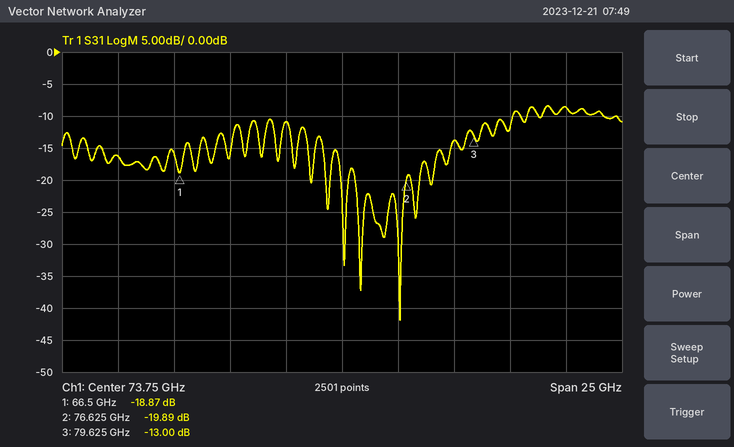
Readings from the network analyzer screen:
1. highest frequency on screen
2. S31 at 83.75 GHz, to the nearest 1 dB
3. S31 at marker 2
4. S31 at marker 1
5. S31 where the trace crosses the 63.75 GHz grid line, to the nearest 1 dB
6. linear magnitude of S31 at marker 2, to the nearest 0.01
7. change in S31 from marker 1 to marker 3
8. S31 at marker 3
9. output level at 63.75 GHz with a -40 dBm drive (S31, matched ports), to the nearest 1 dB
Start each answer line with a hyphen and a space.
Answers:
- 86.25 GHz
- -9 dB
- -19.89 dB
- -18.87 dB
- -16 dB
- 0.10
- 5.87 dB
- -13.00 dB
- -56 dBm
